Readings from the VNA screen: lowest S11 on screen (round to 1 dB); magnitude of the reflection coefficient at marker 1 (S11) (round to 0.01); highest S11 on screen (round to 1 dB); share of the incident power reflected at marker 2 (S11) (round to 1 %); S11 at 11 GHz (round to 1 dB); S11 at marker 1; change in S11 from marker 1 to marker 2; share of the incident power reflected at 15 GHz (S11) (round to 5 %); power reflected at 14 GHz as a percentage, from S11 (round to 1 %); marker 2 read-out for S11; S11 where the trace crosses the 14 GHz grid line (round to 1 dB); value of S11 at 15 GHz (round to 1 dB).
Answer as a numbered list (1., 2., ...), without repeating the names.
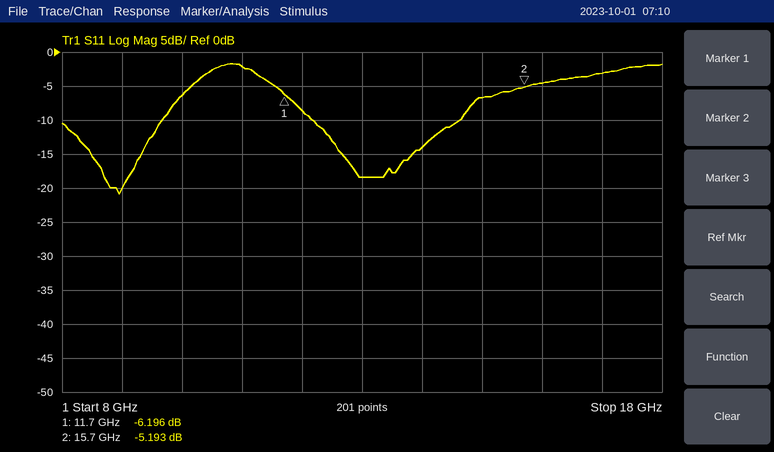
1. -21 dB
2. 0.49
3. -2 dB
4. 30 %
5. -2 dB
6. -6.196 dB
7. 1.003 dB
8. 20 %
9. 4 %
10. -5.193 dB
11. -14 dB
12. -7 dB
